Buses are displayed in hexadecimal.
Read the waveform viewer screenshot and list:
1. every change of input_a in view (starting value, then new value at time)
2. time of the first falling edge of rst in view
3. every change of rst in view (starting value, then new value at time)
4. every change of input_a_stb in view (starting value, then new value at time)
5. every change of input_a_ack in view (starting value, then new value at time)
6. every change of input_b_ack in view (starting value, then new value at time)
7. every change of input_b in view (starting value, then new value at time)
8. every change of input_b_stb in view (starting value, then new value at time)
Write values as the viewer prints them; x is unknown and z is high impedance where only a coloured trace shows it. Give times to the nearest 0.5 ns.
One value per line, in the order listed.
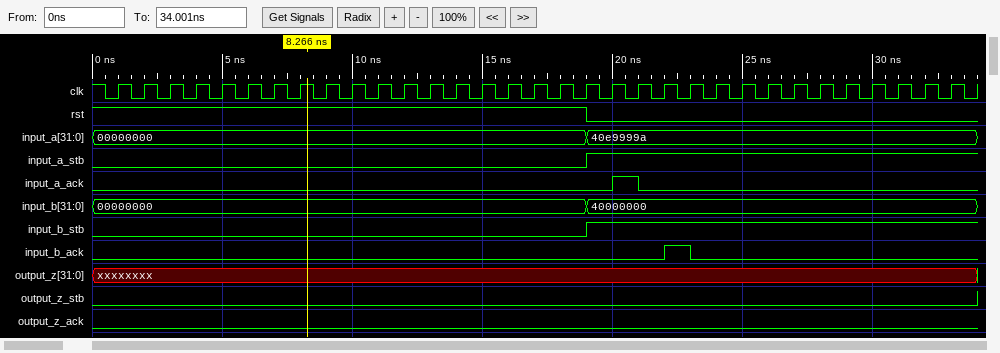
00000000, 40e9999a at 19 ns
19 ns
1, 0 at 19 ns
0, 1 at 19 ns
0, 1 at 20 ns, 0 at 21 ns
0, 1 at 22 ns, 0 at 23 ns
00000000, 40000000 at 19 ns
0, 1 at 19 ns
